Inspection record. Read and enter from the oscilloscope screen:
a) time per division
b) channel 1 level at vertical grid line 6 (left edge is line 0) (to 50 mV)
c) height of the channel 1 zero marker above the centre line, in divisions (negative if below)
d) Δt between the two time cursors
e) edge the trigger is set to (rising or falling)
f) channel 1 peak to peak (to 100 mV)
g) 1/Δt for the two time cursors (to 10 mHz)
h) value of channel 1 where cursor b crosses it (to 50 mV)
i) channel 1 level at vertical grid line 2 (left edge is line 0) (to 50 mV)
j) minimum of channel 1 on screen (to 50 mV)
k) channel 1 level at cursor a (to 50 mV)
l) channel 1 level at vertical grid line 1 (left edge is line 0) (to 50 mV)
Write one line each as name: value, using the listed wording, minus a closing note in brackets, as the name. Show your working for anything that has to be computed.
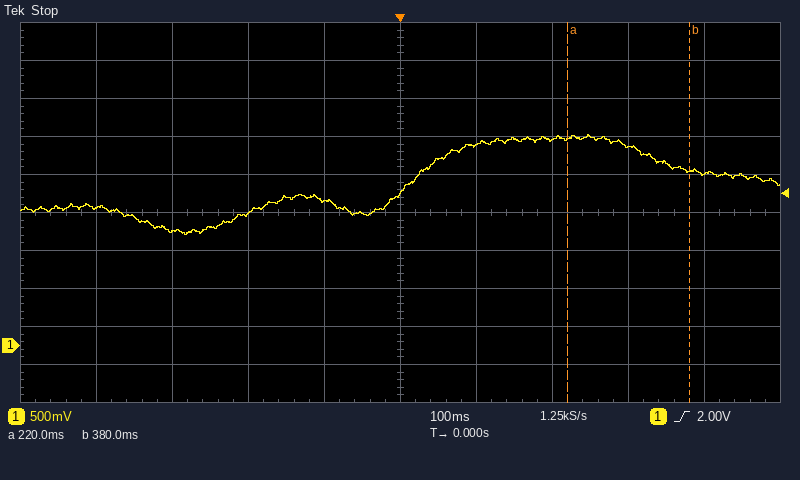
time per division: 100 ms
channel 1 level at vertical grid line 6 (left edge is line 0): 2.65 V
height of the channel 1 zero marker above the centre line, in divisions: -3.5 div
Δt between the two time cursors: 380 ms − (220 ms) = 160 ms
edge the trigger is set to: rising
channel 1 peak to peak: 1.30 V
1/Δt for the two time cursors: 1 / 160 ms ≈ 6.25 Hz
value of channel 1 where cursor b crosses it: 2.30 V
channel 1 level at vertical grid line 2 (left edge is line 0): 1.50 V
minimum of channel 1 on screen: 1.45 V
channel 1 level at cursor a: 2.70 V
channel 1 level at vertical grid line 1 (left edge is line 0): 1.80 V
